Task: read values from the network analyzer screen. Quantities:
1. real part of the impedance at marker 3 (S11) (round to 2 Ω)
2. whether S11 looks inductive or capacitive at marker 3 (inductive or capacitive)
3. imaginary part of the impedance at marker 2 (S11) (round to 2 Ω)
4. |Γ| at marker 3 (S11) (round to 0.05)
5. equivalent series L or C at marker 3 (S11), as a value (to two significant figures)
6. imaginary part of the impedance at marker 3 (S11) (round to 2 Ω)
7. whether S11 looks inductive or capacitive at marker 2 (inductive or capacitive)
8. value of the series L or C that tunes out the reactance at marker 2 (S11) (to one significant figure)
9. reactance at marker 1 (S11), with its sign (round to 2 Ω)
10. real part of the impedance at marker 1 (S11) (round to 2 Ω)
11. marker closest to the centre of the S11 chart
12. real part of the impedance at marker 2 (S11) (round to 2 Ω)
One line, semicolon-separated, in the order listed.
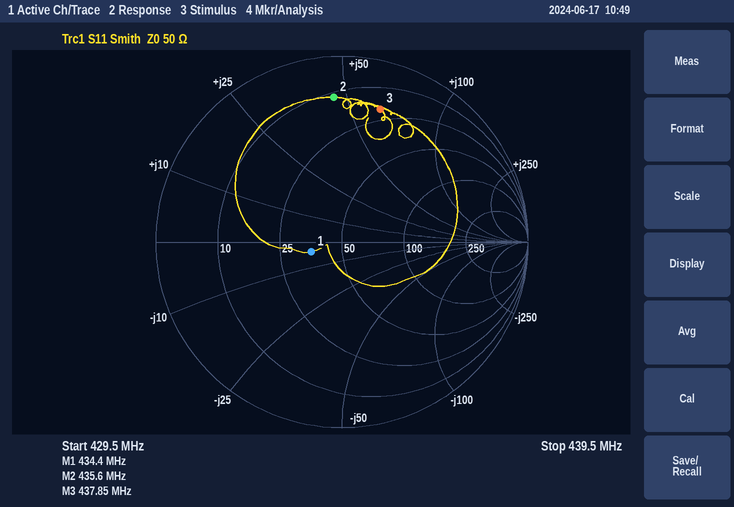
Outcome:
20 Ω; inductive; +46 Ω; 0.75; 23 nH; +62 Ω; inductive; 8 pF; -4 Ω; 36 Ω; marker 1; 12 Ω
